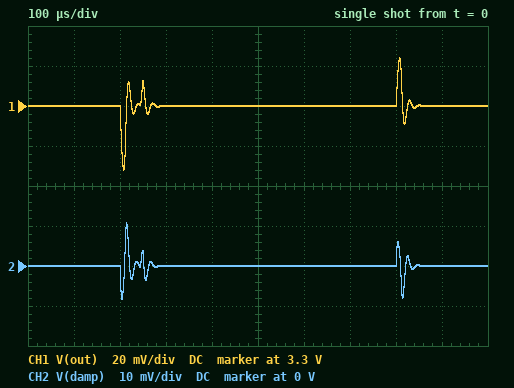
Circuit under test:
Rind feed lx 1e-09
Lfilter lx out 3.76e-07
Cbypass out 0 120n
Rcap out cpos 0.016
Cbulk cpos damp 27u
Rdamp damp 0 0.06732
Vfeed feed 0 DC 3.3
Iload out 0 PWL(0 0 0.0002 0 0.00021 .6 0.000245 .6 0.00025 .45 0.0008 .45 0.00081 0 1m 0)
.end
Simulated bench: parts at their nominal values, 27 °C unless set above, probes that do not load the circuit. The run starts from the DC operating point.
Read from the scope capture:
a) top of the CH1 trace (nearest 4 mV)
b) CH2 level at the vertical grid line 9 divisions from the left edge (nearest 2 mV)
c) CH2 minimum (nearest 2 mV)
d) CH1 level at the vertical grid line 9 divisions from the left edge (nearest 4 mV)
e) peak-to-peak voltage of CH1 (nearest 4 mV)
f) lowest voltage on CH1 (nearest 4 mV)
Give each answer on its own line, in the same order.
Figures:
3.324 V
0 V
-8 mV
3.300 V
56 mV
3.268 V
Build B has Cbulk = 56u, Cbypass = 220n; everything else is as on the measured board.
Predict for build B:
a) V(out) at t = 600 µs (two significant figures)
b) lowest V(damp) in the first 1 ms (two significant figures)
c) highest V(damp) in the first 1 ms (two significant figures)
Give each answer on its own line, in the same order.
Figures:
3.3 V
-10 mV
9.8 mV
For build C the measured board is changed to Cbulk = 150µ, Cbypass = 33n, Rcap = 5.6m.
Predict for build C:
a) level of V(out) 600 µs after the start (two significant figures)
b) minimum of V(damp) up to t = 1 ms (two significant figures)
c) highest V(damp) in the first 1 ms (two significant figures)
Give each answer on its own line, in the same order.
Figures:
3.3 V
-14 mV
10 mV
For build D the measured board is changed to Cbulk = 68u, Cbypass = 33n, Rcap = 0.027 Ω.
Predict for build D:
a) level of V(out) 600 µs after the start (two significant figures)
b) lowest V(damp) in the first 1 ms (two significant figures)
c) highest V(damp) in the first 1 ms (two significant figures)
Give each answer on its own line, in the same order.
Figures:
3.3 V
-9.9 mV
8.1 mV
